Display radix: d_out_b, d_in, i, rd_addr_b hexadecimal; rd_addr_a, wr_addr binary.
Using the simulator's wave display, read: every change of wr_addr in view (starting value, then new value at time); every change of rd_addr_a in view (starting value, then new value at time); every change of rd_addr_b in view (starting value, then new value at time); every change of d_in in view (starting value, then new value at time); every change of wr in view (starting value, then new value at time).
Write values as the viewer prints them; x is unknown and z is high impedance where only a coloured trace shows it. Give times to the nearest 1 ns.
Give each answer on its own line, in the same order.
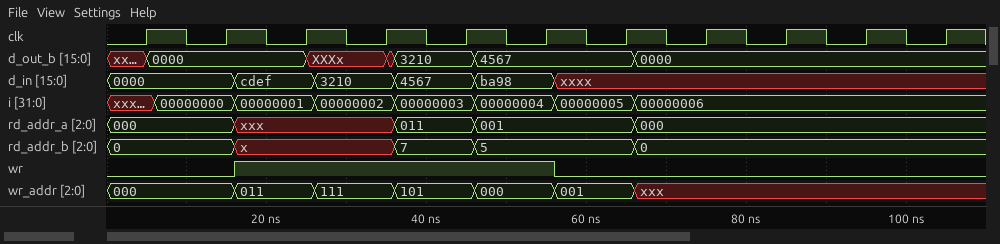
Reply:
000, 011 at 16 ns, 111 at 26 ns, 101 at 36 ns, 000 at 46 ns, 001 at 56 ns, xxx at 66 ns
000, xxx at 16 ns, 011 at 36 ns, 001 at 46 ns, 000 at 66 ns
0, x at 16 ns, 7 at 36 ns, 5 at 46 ns, 0 at 66 ns
0000, cdef at 16 ns, 3210 at 26 ns, 4567 at 36 ns, ba98 at 46 ns, xxxx at 56 ns
0, 1 at 16 ns, 0 at 56 ns
